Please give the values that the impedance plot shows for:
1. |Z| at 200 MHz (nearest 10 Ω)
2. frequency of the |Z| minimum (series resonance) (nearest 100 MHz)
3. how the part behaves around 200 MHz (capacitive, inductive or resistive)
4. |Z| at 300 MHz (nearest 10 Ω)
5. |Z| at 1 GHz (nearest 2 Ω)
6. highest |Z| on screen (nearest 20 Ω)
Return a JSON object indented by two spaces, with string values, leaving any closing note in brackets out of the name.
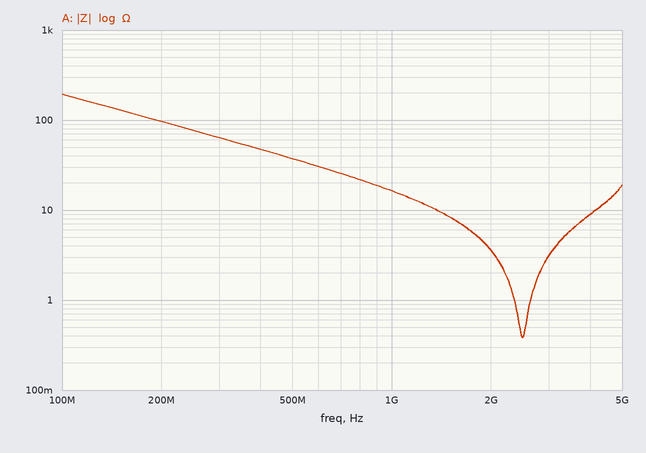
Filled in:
{
  "|Z| at 200 MHz": "100 Ω",
  "frequency of the |Z| minimum (series resonance)": "2.5 GHz",
  "how the part behaves around 200 MHz": "capacitive",
  "|Z| at 300 MHz": "60 Ω",
  "|Z| at 1 GHz": "16 Ω",
  "highest |Z| on screen": "200 Ω"
}
